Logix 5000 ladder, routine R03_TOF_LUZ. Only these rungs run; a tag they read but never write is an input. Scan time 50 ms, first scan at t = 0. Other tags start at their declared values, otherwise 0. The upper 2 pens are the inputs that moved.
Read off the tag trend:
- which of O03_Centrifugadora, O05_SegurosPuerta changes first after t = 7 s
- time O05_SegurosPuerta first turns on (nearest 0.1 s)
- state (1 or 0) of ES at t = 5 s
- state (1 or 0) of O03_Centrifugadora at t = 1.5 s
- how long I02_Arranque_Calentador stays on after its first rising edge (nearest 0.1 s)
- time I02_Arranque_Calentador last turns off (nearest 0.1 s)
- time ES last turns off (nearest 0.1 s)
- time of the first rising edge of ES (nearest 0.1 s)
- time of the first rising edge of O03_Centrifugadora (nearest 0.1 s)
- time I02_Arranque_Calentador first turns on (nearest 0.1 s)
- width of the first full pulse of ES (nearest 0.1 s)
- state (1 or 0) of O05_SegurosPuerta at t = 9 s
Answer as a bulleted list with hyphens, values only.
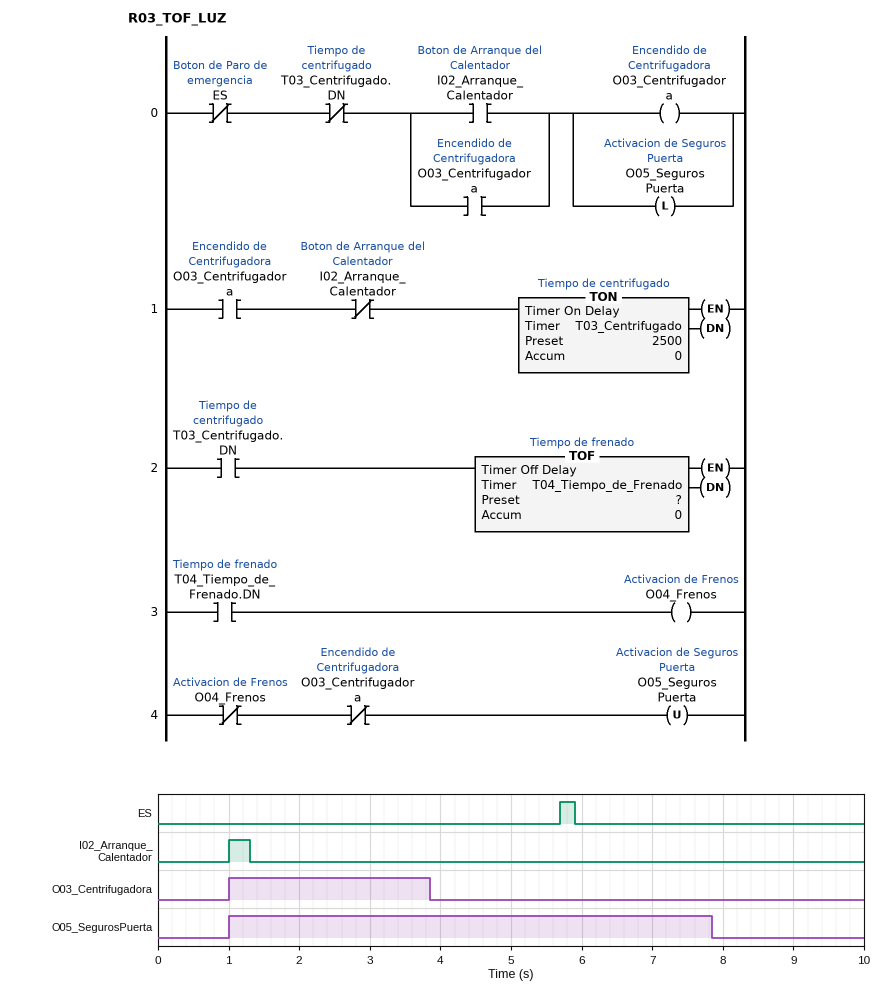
- O05_SegurosPuerta
- 1.0 s
- 0
- 1
- 0.3 s
- 1.3 s
- 5.9 s
- 5.7 s
- 1.0 s
- 1.0 s
- 0.2 s
- 0
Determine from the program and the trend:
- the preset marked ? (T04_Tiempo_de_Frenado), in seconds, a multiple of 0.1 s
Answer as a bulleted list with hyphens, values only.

- 4.0 s
